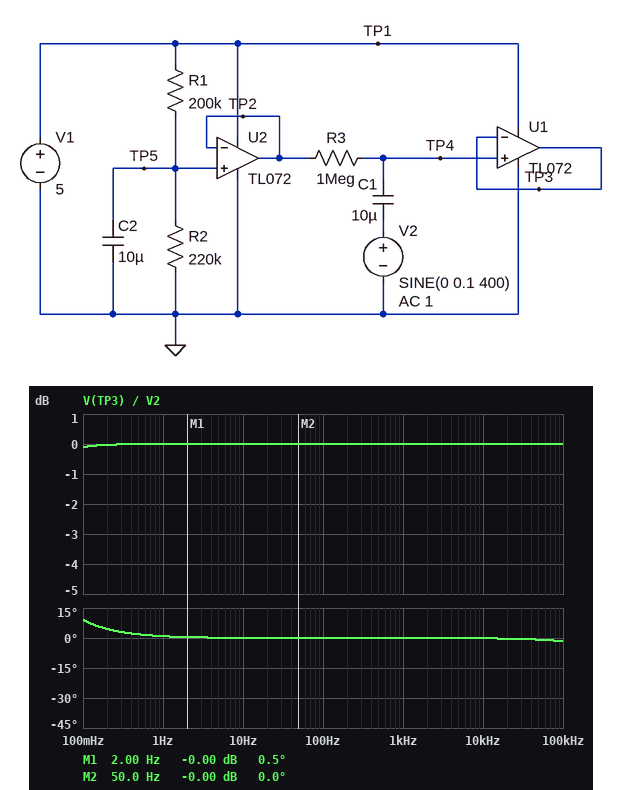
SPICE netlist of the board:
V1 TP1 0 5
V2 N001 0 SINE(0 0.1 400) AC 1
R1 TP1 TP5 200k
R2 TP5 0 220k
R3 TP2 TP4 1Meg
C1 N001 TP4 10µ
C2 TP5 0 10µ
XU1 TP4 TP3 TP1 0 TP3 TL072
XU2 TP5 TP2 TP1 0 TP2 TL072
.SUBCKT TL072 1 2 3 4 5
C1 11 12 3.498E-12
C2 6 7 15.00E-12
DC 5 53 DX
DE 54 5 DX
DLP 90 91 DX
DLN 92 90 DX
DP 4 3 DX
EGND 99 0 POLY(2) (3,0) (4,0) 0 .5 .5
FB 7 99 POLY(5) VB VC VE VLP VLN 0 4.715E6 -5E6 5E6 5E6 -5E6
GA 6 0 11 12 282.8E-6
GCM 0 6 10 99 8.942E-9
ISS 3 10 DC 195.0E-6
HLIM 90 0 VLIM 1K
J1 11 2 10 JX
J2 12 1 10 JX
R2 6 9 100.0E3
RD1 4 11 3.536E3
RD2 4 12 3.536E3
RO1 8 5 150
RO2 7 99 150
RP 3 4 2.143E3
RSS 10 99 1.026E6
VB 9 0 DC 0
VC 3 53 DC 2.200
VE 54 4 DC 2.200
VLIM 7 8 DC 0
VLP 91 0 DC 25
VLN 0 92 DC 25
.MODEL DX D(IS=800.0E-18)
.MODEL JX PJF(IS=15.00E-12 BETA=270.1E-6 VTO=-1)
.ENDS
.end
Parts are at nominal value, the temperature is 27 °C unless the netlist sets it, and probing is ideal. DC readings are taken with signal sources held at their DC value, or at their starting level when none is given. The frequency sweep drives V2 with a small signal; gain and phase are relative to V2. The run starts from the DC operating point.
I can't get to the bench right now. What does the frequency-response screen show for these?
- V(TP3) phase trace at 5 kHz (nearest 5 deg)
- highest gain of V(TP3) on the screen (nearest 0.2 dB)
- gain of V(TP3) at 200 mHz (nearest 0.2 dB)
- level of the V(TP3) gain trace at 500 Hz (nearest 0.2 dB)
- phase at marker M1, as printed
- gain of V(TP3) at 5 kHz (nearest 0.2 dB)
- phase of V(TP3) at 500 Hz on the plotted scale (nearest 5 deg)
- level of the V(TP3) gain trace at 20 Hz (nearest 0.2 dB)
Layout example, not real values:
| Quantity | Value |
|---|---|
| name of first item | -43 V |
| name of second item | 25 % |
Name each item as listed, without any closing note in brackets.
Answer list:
| Quantity | Value |
|---|---|
| V(TP3) phase trace at 5 kHz | 0 deg |
| highest gain of V(TP3) on the screen | 0 dB |
| gain of V(TP3) at 200 mHz | 0 dB |
| level of the V(TP3) gain trace at 500 Hz | 0 dB |
| phase at marker M1, as printed | 0.5 deg |
| gain of V(TP3) at 5 kHz | 0 dB |
| phase of V(TP3) at 500 Hz on the plotted scale | 0 deg |
| level of the V(TP3) gain trace at 20 Hz | 0 dB |
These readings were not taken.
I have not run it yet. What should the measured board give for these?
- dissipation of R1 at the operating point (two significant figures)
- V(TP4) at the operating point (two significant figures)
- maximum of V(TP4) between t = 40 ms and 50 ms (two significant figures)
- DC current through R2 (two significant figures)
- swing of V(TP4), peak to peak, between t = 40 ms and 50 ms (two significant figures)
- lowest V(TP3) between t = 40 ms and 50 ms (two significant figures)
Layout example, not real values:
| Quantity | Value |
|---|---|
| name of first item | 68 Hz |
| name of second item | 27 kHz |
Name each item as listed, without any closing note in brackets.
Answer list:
| Quantity | Value |
|---|---|
| dissipation of R1 at the operating point | 28 µW |
| V(TP4) at the operating point | 2.6 V |
| maximum of V(TP4) between t = 40 ms and 50 ms | 2.7 V |
| DC current through R2 | 12 µA |
| swing of V(TP4), peak to peak, between t = 40 ms and 50 ms | 200 mV |
| lowest V(TP3) between t = 40 ms and 50 ms | 2.5 V |
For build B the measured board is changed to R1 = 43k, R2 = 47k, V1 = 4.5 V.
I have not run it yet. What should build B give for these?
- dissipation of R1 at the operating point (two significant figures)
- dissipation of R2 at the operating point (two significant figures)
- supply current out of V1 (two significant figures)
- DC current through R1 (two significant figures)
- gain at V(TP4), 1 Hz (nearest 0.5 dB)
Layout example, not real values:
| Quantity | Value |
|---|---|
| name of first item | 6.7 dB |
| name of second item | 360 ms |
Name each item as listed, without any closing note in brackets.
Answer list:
| Quantity | Value |
|---|---|
| dissipation of R1 at the operating point | 110 µW |
| dissipation of R2 at the operating point | 120 µW |
| supply current out of V1 | 4.6 mA |
| DC current through R1 | 50 µA |
| gain at V(TP4), 1 Hz | 0 dB |
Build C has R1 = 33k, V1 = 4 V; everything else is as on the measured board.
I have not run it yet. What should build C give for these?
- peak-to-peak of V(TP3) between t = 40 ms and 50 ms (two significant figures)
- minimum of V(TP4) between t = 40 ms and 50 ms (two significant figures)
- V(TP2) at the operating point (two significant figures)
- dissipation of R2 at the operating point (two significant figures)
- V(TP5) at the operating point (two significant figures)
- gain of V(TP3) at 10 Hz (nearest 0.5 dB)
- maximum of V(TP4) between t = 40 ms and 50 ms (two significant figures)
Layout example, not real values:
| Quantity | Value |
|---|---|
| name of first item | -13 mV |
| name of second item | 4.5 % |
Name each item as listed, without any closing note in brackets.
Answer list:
| Quantity | Value |
|---|---|
| peak-to-peak of V(TP3) between t = 40 ms and 50 ms | 71 mV |
| minimum of V(TP4) between t = 40 ms and 50 ms | 2.4 V |
| V(TP2) at the operating point | 2.5 V |
| dissipation of R2 at the operating point | 55 µW |
| V(TP5) at the operating point | 3.5 V |
| gain of V(TP3) at 10 Hz | -10.5 dB |
| maximum of V(TP4) between t = 40 ms and 50 ms | 2.6 V |
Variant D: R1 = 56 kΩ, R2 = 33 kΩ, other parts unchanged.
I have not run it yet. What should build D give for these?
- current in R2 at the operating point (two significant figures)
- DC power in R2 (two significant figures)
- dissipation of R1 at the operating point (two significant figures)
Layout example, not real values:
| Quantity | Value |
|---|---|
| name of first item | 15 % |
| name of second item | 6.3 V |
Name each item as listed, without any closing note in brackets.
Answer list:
| Quantity | Value |
|---|---|
| current in R2 at the operating point | 56 µA |
| DC power in R2 | 100 µW |
| dissipation of R1 at the operating point | 180 µW |
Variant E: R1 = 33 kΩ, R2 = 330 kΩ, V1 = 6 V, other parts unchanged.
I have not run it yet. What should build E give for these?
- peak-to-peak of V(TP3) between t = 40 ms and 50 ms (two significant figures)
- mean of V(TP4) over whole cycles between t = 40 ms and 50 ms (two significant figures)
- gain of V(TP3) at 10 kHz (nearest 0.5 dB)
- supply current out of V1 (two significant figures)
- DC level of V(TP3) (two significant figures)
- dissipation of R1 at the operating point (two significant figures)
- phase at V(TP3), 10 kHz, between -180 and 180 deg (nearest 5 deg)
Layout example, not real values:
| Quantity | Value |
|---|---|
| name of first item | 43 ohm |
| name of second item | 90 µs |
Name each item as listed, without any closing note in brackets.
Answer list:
| Quantity | Value |
|---|---|
| peak-to-peak of V(TP3) between t = 40 ms and 50 ms | 71 mV |
| mean of V(TP4) over whole cycles between t = 40 ms and 50 ms | 4.5 V |
| gain of V(TP3) at 10 kHz | -10.5 dB |
| supply current out of V1 | 5.8 mA |
| DC level of V(TP3) | 4.4 V |
| dissipation of R1 at the operating point | 9.0 µW |
| phase at V(TP3), 10 kHz, between -180 and 180 deg | -5 deg |
